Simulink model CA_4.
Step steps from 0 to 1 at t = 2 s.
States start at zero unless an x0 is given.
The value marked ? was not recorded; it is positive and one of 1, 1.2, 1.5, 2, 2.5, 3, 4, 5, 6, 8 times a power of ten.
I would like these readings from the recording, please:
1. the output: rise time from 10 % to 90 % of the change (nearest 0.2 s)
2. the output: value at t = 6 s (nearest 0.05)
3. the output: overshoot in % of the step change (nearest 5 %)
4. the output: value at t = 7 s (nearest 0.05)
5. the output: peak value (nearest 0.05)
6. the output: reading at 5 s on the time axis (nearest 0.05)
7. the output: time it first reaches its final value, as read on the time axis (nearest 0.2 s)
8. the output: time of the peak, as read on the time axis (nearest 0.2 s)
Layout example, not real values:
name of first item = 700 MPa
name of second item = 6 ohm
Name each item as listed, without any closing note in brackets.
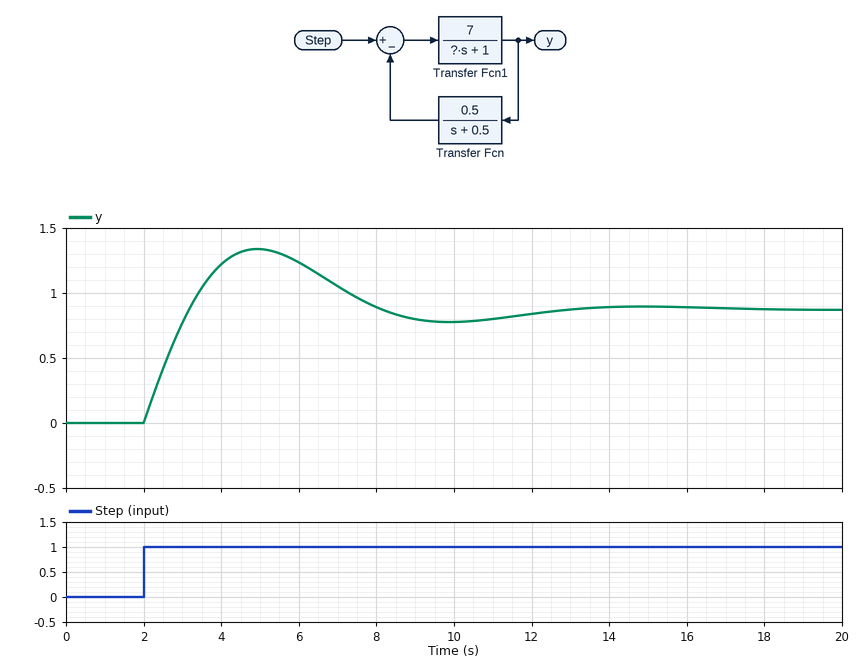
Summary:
the output: rise time from 10 % to 90 % of the change = 1.0 s
the output: value at t = 6 s = 1.25
the output: overshoot in % of the step change = 55 %
the output: value at t = 7 s = 1.05
the output: peak value = 1.35
the output: reading at 5 s on the time axis = 1.35
the output: time it first reaches its final value, as read on the time axis = 3.2 s
the output: time of the peak, as read on the time axis = 5.0 s
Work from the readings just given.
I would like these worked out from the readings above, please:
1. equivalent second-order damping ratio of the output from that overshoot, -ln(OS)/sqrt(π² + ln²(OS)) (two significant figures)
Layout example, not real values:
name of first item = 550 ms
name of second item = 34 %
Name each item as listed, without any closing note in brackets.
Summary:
equivalent second-order damping ratio of the output from that overshoot, -ln(OS)/sqrt(π² + ln²(OS)) = 0.19
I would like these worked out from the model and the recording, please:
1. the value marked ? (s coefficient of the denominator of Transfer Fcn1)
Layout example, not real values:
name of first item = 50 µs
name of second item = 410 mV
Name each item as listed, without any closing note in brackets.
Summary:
the value marked ? = 8
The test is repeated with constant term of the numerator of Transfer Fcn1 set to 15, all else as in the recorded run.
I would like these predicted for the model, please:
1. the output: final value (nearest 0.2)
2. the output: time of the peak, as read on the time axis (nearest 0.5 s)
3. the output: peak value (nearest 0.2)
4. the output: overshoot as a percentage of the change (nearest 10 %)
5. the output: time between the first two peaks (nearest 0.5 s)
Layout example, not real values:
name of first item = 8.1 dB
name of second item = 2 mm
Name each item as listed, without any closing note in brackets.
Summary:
the output: final value = 1.0
the output: time of the peak, as read on the time axis = 4.0 s
the output: peak value = 2.0
the output: overshoot as a percentage of the change = 110 %
the output: time between the first two peaks = 6.5 s
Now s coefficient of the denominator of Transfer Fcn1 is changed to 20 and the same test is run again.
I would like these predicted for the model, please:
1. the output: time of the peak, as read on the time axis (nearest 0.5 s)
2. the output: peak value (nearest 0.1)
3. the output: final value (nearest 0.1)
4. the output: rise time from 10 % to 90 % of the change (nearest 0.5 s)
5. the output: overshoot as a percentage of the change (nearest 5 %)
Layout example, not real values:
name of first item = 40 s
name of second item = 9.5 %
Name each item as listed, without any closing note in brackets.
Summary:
the output: time of the peak, as read on the time axis = 8.0 s
the output: peak value = 1.0
the output: final value = 0.9
the output: rise time from 10 % to 90 % of the change = 2.5 s
the output: overshoot as a percentage of the change = 15 %
